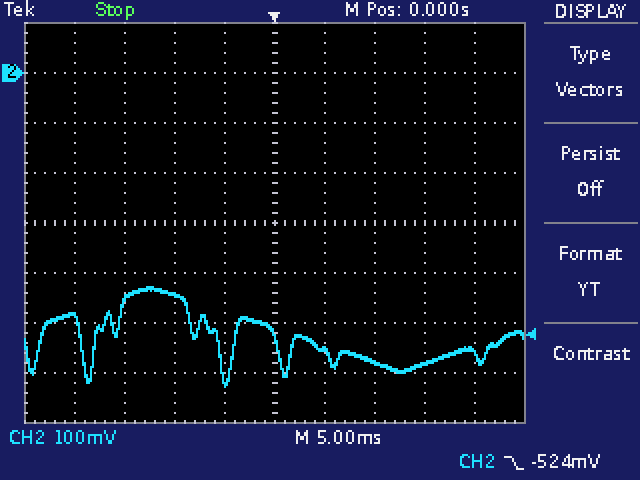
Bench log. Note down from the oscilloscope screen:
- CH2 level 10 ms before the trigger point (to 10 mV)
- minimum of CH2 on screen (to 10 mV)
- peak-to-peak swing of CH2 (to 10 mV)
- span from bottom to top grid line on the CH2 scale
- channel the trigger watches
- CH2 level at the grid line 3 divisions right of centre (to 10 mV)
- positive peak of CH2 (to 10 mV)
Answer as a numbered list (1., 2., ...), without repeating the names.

1. -440 mV
2. -630 mV
3. 200 mV
4. 800 mV
5. CH2
6. -580 mV
7. -430 mV
